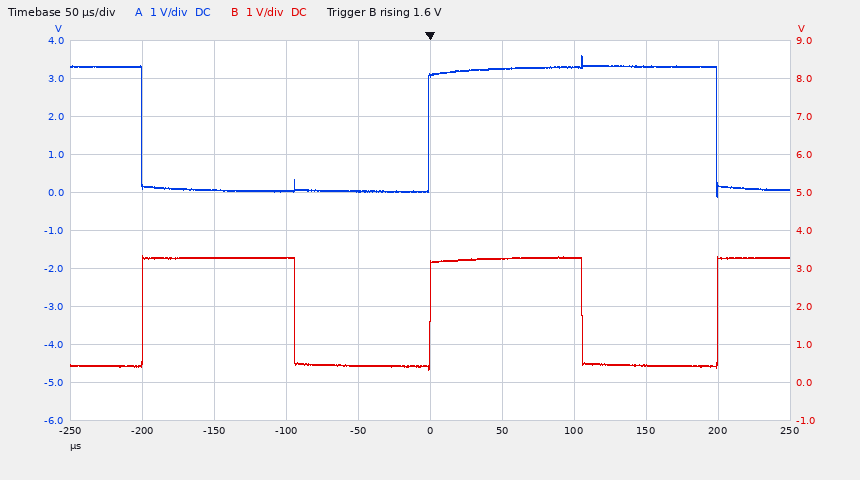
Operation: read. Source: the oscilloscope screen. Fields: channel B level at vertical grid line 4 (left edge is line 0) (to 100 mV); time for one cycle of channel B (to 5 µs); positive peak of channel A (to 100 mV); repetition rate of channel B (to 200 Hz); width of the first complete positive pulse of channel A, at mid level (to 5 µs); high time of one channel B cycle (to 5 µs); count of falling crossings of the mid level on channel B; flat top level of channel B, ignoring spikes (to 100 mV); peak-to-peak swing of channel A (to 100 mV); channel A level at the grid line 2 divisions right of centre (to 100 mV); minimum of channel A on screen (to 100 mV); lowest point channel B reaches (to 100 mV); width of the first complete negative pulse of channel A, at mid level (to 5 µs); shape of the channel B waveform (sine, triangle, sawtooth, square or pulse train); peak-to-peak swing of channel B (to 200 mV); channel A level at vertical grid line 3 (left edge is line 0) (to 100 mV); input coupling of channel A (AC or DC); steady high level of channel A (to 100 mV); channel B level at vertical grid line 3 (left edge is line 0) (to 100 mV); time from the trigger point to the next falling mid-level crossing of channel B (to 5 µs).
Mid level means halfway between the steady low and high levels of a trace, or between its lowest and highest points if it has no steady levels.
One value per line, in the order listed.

400 mV
200 µs
3.6 V
5.0 kHz
200 µs
105 µs
2
3.3 V
3.7 V
3.3 V
-100 mV
300 mV
200 µs
square
3.0 V
0.0 V
DC
3.3 V
3.3 V
105 µs
